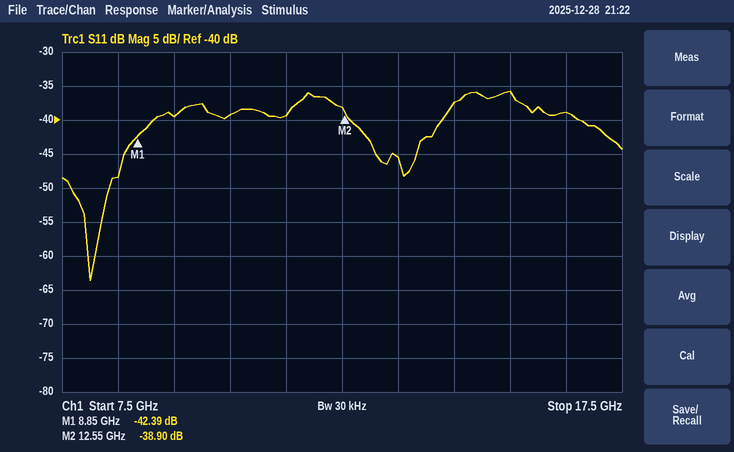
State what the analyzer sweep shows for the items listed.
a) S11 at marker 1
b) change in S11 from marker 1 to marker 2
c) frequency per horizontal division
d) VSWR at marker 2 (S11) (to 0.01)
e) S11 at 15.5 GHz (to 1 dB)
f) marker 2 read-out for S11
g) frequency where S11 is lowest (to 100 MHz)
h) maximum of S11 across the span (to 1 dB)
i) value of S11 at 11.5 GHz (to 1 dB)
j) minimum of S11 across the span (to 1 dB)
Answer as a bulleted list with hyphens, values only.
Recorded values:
- -42.39 dB
- 3.49 dB
- 1 GHz
- 1.02
- -36 dB
- -38.90 dB
- 8.0 GHz
- -36 dB
- -39 dB
- -64 dB
